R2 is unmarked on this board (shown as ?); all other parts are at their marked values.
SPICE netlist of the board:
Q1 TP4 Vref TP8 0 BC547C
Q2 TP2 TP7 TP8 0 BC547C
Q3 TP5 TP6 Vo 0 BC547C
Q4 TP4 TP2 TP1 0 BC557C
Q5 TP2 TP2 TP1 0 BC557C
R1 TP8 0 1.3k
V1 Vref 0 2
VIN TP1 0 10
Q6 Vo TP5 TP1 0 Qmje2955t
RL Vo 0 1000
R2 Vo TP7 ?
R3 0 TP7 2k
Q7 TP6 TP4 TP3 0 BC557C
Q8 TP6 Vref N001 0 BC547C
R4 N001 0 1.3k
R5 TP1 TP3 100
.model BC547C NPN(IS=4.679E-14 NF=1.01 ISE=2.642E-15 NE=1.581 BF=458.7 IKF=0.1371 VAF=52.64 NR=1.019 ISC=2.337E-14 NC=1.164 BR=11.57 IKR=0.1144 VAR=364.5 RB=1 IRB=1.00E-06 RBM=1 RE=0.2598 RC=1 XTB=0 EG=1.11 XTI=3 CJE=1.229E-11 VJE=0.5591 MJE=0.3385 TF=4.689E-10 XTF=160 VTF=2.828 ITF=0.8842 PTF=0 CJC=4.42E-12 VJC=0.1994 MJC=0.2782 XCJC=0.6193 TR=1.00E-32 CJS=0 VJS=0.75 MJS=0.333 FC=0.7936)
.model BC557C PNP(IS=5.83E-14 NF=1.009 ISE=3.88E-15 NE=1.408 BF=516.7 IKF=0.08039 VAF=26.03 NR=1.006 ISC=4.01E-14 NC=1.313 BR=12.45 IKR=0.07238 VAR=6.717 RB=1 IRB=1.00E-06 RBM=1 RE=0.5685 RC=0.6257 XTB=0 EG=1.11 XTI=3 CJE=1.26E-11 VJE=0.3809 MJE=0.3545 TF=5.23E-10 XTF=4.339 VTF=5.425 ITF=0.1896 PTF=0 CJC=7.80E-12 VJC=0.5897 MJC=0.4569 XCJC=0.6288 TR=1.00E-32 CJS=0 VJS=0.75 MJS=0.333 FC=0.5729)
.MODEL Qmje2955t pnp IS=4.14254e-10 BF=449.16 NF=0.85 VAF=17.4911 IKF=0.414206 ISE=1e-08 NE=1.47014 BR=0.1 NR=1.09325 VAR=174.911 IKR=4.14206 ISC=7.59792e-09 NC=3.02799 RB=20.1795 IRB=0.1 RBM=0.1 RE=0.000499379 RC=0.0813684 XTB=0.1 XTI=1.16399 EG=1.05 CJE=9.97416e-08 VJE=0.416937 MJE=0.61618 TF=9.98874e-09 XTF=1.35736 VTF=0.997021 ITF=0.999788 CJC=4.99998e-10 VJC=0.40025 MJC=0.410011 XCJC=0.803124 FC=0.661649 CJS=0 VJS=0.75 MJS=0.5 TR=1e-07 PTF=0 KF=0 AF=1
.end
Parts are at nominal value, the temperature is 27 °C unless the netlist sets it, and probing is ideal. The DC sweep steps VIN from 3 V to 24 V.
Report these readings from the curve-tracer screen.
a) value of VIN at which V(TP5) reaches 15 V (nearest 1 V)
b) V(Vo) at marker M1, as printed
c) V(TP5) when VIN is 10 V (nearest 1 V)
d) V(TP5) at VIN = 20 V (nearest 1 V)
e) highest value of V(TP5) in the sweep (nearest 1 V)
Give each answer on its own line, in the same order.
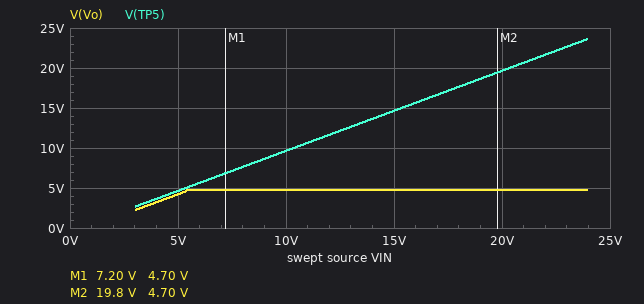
15 V
4.70 V
10 V
20 V
24 V
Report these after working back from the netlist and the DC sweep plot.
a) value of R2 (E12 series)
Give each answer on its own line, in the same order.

2.7 kΩ
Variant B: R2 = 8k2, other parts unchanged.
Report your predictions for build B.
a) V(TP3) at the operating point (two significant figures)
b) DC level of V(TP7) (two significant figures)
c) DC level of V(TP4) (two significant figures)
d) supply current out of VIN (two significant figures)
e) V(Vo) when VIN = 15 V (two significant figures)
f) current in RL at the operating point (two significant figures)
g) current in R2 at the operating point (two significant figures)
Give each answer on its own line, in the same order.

9.8 V
1.8 V
9.1 V
12 mA
10 V
9.2 mA
900 µA
